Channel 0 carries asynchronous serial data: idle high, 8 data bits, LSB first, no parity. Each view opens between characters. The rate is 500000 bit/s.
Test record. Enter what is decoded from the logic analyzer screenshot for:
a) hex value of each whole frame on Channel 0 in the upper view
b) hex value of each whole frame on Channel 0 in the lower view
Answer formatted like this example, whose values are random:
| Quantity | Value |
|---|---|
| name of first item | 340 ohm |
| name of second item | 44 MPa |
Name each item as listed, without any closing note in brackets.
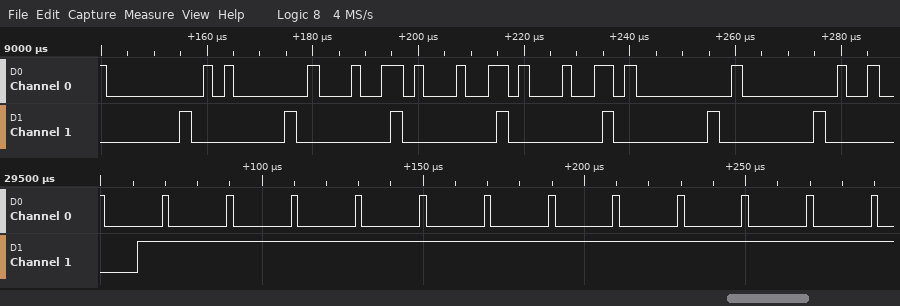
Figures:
| Quantity | Value |
|---|---|
| hex value of each whole frame on Channel 0 in the upper view | 00, 01, 64, 64, 64, 00, 00 |
| hex value of each whole frame on Channel 0 in the lower view | 00, 00, 00, 00, 00, 00, 00, 00, 00, 00, 00, 00 |
